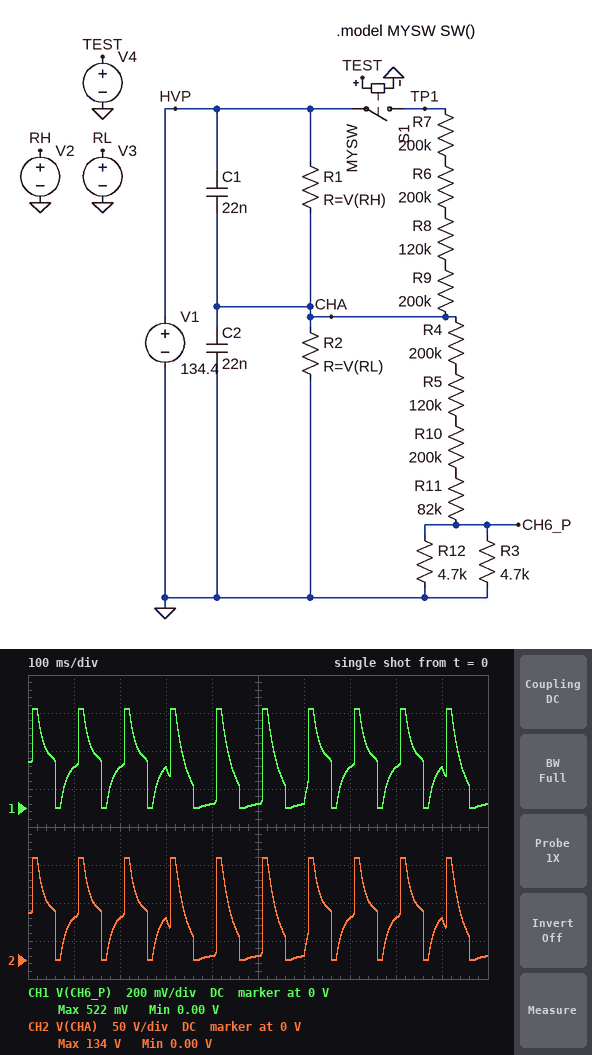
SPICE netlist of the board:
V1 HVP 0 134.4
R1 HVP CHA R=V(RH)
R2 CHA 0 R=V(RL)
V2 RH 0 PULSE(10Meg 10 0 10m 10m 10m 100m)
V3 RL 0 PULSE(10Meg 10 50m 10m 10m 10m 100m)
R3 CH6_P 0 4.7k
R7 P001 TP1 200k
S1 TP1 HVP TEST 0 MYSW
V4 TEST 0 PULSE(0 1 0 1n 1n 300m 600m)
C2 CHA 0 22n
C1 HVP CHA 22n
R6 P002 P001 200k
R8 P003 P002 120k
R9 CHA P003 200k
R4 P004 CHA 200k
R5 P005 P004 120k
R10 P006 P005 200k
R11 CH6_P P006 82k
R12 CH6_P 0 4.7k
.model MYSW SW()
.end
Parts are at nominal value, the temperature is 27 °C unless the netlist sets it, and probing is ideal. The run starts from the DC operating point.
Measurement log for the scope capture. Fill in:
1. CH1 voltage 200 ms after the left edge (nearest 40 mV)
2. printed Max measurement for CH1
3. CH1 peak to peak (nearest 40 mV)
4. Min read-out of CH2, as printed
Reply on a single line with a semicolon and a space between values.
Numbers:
200 mV; 522 mV; 520 mV; 0.00 V
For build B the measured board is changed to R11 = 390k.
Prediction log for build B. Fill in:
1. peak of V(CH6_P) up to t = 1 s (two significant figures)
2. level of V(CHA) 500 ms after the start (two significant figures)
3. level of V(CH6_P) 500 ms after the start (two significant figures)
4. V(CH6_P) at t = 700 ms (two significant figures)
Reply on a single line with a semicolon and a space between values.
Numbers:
350 mV; 6.1 V; 16 mV; 160 mV
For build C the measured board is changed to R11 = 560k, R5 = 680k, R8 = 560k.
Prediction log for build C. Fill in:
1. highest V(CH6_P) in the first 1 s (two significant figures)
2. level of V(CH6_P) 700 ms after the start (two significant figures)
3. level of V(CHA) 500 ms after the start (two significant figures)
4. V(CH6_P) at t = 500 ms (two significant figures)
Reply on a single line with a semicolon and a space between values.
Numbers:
190 mV; 75 mV; 7.0 V; 10 mV
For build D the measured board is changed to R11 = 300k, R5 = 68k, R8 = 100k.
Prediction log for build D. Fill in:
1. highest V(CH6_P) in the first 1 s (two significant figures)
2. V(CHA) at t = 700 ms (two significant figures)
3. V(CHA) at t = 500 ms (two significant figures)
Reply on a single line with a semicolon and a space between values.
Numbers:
410 mV; 61 V; 5.7 V
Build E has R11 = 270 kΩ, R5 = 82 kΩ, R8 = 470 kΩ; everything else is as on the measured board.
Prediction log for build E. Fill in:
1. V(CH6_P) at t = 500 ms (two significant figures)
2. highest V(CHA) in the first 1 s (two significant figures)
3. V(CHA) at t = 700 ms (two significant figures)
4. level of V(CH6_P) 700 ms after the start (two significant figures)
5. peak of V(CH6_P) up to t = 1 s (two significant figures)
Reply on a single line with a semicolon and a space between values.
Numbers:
18 mV; 130 V; 46 V; 140 mV; 420 mV
